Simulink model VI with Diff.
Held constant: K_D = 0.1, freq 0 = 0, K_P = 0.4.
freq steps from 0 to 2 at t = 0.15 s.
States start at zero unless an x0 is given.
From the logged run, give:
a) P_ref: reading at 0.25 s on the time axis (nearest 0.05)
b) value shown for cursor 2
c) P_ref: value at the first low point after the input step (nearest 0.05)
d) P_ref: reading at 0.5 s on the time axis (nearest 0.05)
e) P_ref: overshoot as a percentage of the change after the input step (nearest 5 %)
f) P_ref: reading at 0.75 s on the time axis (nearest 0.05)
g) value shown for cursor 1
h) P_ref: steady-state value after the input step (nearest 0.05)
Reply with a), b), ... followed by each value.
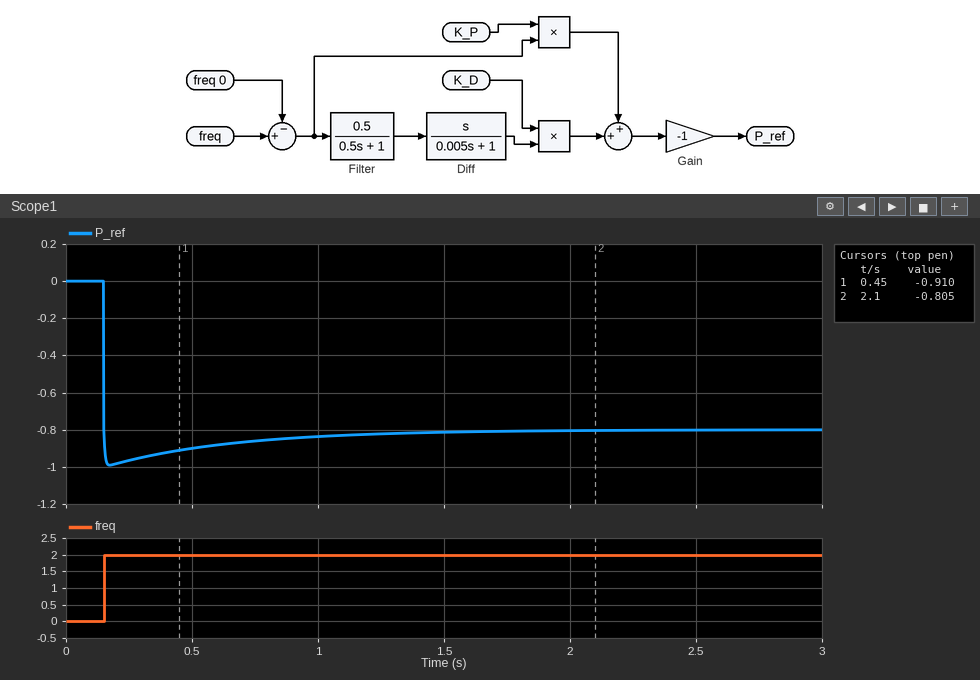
a) -0.95
b) -0.805
c) -1.00
d) -0.90
e) 25 %
f) -0.85
g) -0.910
h) -0.80
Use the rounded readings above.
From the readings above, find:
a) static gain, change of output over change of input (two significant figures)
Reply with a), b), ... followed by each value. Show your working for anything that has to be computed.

a) (-0.8 - 0) / (2 - 0) = -0.40
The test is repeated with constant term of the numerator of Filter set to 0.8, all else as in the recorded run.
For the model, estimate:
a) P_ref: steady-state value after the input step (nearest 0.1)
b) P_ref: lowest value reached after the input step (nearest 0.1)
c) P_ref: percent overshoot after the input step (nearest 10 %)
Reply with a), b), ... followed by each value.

a) -0.8
b) -1.1
c) 40 %
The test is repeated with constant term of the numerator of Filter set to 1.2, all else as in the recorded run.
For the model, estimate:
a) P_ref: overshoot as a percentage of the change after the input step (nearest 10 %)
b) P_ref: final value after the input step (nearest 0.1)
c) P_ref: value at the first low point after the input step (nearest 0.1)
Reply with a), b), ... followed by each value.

a) 60 %
b) -0.8
c) -1.3
